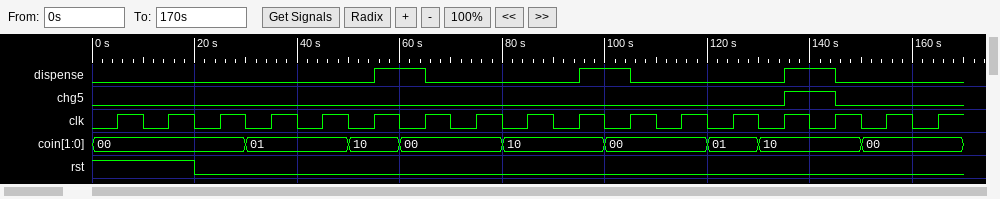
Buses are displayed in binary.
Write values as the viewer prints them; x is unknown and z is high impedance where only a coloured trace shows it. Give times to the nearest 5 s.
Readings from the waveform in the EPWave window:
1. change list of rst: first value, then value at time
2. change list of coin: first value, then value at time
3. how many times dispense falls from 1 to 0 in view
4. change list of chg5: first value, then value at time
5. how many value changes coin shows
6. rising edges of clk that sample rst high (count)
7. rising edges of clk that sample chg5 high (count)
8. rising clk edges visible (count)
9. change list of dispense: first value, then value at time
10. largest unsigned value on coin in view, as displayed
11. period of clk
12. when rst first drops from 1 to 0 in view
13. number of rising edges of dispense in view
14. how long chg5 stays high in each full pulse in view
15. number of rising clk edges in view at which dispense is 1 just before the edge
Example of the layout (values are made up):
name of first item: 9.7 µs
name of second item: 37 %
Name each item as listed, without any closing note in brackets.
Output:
change list of rst: first value, then value at time: 1, 0 at 20 s
change list of coin: first value, then value at time: 00, 01 at 30 s, 10 at 50 s, 00 at 60 s, 10 at 80 s, 00 at 100 s, 01 at 120 s, 10 at 130 s, 00 at 150 s
how many times dispense falls from 1 to 0 in view: 3
change list of chg5: first value, then value at time: 0, 1 at 135 s, 0 at 145 s
how many value changes coin shows: 8
rising edges of clk that sample rst high: 2
rising edges of clk that sample chg5 high: 1
rising clk edges visible: 17
change list of dispense: first value, then value at time: 0, 1 at 55 s, 0 at 65 s, 1 at 95 s, 0 at 105 s, 1 at 135 s, 0 at 145 s
largest unsigned value on coin in view, as displayed: 10
period of clk: 10 s
when rst first drops from 1 to 0 in view: 20 s
number of rising edges of dispense in view: 3
how long chg5 stays high in each full pulse in view: 10 s
number of rising clk edges in view at which dispense is 1 just before the edge: 3
